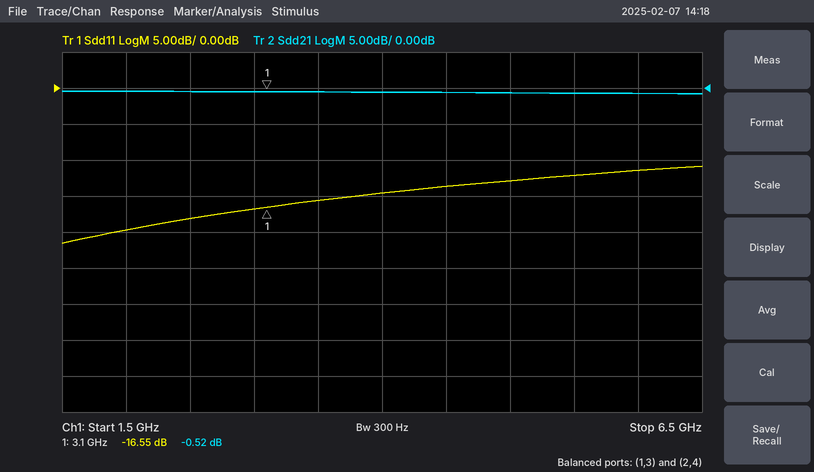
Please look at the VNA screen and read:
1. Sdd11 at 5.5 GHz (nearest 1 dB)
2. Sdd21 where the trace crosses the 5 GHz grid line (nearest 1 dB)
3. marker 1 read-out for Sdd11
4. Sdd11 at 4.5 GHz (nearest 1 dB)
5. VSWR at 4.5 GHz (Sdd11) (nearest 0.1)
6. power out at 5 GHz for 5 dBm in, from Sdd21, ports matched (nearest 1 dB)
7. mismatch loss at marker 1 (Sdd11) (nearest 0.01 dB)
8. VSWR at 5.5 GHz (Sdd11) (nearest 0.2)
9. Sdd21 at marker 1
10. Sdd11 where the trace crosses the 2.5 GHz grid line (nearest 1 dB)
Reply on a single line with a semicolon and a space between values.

-12 dB; -1 dB; -16.55 dB; -14 dB; 1.5; 4 dBm; 0.10 dB; 1.6; -0.52 dB; -18 dB
